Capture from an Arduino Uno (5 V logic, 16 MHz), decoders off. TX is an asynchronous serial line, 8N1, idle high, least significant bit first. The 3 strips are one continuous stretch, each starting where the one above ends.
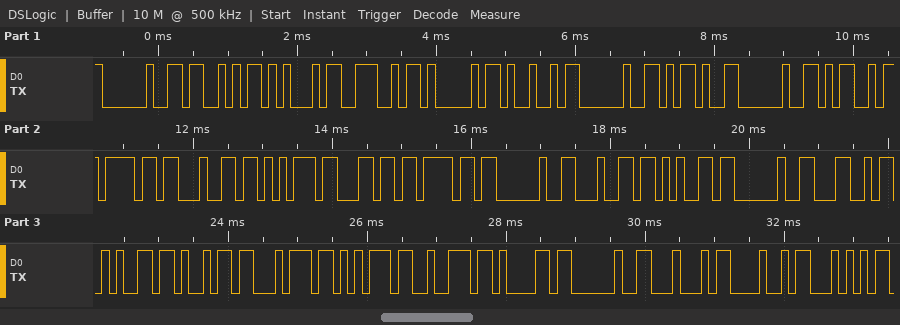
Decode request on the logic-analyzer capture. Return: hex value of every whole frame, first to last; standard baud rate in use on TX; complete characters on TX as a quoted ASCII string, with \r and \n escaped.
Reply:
20 53 45 4E 41 49 20 2D 20 4D 6F 64 75 6C 6F 20 64 65 20 4C 65 69 74 75 72 61 20 44 48 54
9600 baud
" SENAI - Modulo de Leitura DHT"
